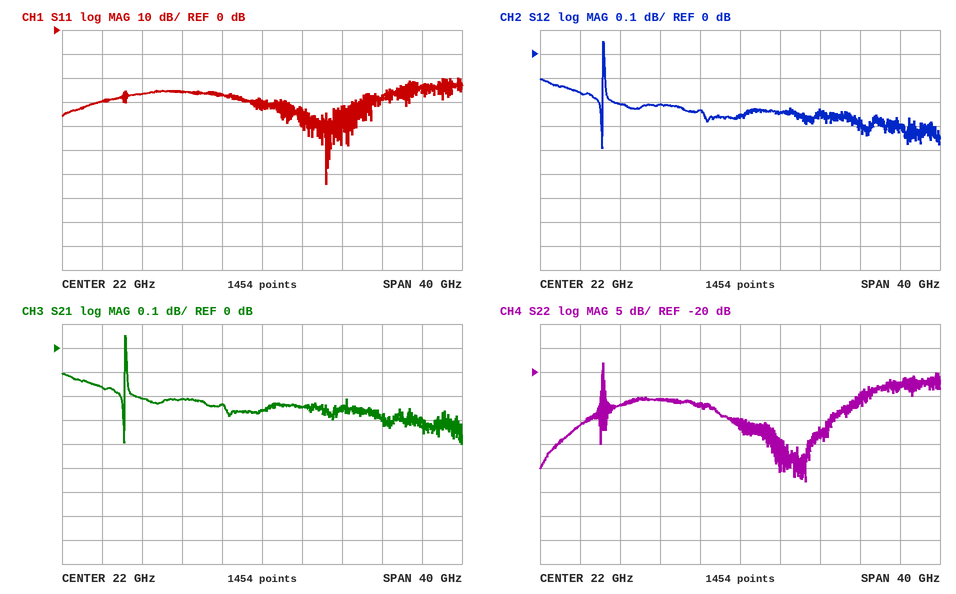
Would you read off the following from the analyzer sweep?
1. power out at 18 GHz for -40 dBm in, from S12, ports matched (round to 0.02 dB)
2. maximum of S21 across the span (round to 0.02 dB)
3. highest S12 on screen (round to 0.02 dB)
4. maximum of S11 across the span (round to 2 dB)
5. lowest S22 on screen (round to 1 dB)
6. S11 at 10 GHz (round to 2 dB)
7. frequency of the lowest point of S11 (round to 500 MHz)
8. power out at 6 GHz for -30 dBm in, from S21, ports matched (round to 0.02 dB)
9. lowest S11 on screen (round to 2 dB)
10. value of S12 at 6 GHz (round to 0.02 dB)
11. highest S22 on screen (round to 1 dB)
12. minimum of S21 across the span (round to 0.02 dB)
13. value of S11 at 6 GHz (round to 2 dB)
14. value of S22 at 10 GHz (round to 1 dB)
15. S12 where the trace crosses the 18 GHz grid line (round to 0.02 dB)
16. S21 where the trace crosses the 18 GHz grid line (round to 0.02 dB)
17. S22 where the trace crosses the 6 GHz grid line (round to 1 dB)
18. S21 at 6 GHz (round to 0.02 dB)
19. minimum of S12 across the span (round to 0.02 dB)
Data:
-40.24 dBm
0.06 dB
0.06 dB
-20 dB
-43 dB
-26 dB
28.5 GHz
-30.16 dBm
-64 dB
-0.16 dB
-18 dB
-0.40 dB
-30 dB
-27 dB
-0.24 dB
-0.24 dB
-31 dB
-0.16 dB
-0.40 dB
